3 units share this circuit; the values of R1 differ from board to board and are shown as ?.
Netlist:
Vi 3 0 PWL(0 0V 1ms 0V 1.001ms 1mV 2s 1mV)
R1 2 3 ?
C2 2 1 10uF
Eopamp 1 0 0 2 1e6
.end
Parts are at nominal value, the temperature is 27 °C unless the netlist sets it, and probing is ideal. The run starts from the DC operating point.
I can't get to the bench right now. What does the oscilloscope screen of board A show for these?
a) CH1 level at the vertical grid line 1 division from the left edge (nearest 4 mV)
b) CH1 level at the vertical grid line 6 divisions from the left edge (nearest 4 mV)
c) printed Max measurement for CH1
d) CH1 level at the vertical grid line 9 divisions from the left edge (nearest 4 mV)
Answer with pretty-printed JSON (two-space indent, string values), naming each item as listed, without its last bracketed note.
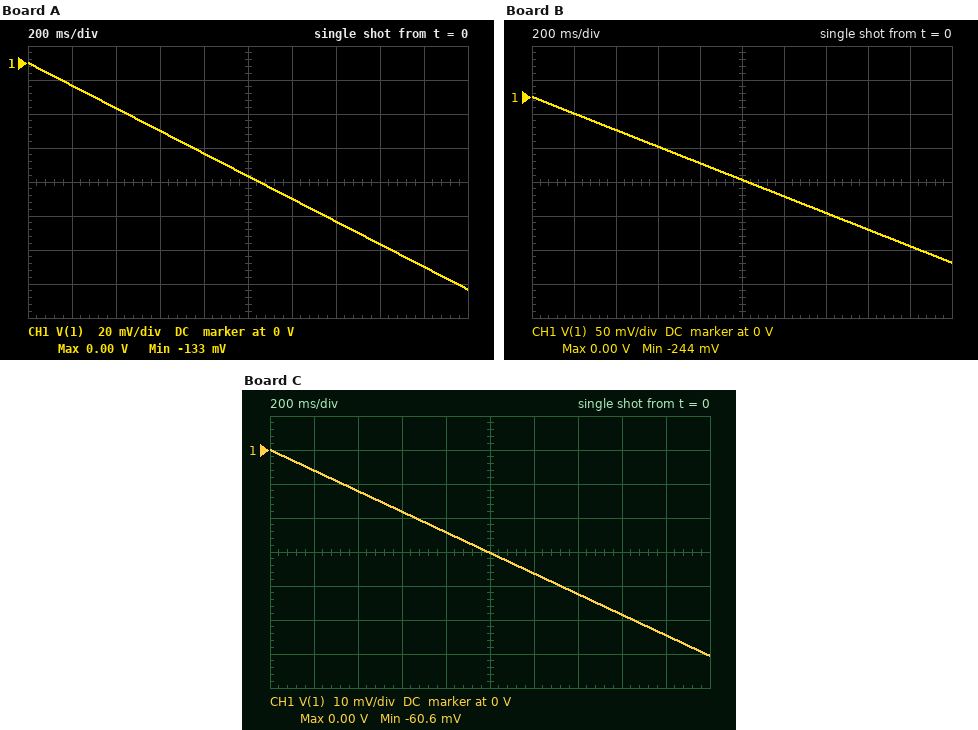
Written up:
{
  "CH1 level at the vertical grid line 1 division from the left edge": "-12 mV",
  "CH1 level at the vertical grid line 6 divisions from the left edge": "-80 mV",
  "printed Max measurement for CH1": "0.00 V",
  "CH1 level at the vertical grid line 9 divisions from the left edge": "-120 mV"
}
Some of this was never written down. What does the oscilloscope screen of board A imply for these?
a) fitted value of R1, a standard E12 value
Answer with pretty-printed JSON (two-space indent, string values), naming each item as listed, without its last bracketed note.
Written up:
{
  "fitted value of R1, a standard E12 value": "1.5 kΩ"
}
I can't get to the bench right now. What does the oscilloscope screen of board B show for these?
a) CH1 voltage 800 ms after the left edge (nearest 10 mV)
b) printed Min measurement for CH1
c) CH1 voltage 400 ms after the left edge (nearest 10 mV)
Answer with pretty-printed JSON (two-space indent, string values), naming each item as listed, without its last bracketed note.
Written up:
{
  "CH1 voltage 800 ms after the left edge": "-100 mV",
  "printed Min measurement for CH1": "-244 mV",
  "CH1 voltage 400 ms after the left edge": "-50 mV"
}
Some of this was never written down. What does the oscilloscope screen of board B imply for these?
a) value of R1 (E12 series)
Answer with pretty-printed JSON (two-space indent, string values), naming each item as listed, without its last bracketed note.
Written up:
{
  "value of R1": "820 Ω"
}
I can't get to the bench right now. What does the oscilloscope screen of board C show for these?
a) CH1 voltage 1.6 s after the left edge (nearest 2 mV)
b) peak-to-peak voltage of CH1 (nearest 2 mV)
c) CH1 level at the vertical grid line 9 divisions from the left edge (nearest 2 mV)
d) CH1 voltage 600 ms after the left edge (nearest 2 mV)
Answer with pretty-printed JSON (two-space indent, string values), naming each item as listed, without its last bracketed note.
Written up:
{
  "CH1 voltage 1.6 s after the left edge": "-48 mV",
  "peak-to-peak voltage of CH1": "60 mV",
  "CH1 level at the vertical grid line 9 divisions from the left edge": "-54 mV",
  "CH1 voltage 600 ms after the left edge": "-18 mV"
}
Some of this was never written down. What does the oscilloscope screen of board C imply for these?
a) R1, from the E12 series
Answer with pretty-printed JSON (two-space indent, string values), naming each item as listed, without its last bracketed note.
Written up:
{
  "R1, from the E12 series": "3.3 kΩ"
}
